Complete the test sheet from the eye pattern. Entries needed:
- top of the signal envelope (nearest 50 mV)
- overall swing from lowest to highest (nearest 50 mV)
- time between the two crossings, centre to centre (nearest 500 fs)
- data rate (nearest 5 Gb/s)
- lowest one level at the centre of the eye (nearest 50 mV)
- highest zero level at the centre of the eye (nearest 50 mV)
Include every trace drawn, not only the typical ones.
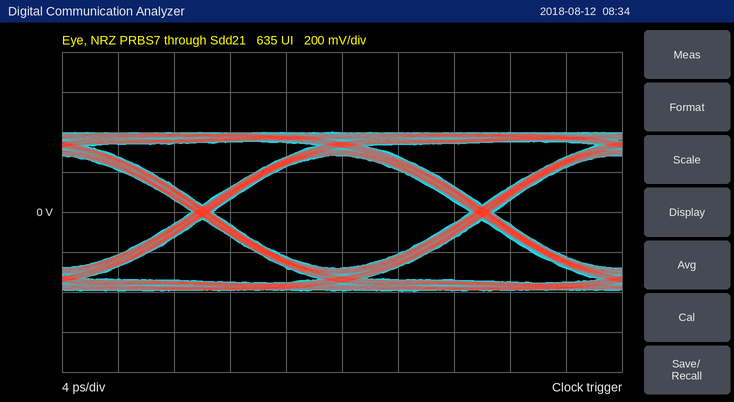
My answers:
400 mV
800 mV
20.0 ps
50 Gb/s
300 mV
-300 mV
